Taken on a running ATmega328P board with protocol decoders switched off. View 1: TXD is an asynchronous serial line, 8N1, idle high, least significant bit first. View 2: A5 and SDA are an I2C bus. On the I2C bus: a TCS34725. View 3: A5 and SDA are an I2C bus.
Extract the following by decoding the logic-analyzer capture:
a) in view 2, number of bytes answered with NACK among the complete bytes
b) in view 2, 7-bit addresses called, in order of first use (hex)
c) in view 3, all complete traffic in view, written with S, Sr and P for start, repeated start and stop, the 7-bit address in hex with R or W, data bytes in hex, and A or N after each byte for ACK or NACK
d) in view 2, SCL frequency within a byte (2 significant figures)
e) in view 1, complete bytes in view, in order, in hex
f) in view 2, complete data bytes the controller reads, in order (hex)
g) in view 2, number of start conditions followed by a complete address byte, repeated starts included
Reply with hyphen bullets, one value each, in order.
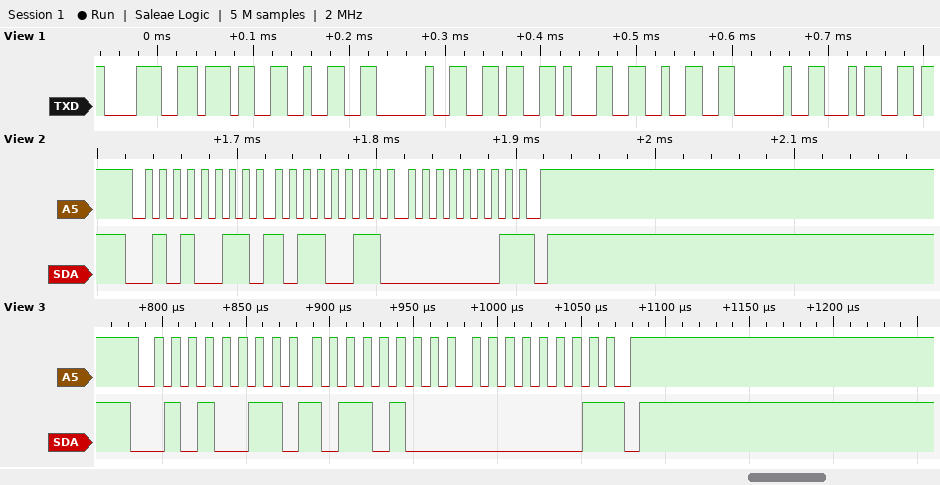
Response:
- 1
- 0x29
- S 29R A B4 A 01 N P
- 100 kHz
- 38 37 32 20 36 31 32 20 34
- B3 01
- 1
